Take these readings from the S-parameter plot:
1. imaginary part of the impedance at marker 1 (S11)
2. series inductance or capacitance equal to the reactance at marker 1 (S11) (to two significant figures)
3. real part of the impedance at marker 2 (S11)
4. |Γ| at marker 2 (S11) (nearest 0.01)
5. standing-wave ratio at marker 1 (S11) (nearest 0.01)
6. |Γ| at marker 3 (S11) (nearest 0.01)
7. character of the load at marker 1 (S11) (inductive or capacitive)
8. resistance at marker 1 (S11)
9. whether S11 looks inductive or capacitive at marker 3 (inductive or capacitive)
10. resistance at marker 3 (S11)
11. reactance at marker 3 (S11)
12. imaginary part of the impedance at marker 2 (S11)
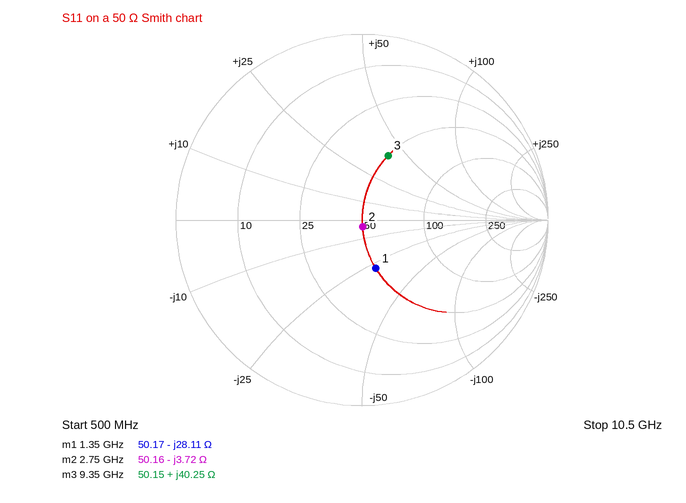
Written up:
-28.11 Ω
4.2 pF
50.16 Ω
0.04
1.74
0.37
capacitive
50.17 Ω
inductive
50.15 Ω
+40.25 Ω
-3.72 Ω
